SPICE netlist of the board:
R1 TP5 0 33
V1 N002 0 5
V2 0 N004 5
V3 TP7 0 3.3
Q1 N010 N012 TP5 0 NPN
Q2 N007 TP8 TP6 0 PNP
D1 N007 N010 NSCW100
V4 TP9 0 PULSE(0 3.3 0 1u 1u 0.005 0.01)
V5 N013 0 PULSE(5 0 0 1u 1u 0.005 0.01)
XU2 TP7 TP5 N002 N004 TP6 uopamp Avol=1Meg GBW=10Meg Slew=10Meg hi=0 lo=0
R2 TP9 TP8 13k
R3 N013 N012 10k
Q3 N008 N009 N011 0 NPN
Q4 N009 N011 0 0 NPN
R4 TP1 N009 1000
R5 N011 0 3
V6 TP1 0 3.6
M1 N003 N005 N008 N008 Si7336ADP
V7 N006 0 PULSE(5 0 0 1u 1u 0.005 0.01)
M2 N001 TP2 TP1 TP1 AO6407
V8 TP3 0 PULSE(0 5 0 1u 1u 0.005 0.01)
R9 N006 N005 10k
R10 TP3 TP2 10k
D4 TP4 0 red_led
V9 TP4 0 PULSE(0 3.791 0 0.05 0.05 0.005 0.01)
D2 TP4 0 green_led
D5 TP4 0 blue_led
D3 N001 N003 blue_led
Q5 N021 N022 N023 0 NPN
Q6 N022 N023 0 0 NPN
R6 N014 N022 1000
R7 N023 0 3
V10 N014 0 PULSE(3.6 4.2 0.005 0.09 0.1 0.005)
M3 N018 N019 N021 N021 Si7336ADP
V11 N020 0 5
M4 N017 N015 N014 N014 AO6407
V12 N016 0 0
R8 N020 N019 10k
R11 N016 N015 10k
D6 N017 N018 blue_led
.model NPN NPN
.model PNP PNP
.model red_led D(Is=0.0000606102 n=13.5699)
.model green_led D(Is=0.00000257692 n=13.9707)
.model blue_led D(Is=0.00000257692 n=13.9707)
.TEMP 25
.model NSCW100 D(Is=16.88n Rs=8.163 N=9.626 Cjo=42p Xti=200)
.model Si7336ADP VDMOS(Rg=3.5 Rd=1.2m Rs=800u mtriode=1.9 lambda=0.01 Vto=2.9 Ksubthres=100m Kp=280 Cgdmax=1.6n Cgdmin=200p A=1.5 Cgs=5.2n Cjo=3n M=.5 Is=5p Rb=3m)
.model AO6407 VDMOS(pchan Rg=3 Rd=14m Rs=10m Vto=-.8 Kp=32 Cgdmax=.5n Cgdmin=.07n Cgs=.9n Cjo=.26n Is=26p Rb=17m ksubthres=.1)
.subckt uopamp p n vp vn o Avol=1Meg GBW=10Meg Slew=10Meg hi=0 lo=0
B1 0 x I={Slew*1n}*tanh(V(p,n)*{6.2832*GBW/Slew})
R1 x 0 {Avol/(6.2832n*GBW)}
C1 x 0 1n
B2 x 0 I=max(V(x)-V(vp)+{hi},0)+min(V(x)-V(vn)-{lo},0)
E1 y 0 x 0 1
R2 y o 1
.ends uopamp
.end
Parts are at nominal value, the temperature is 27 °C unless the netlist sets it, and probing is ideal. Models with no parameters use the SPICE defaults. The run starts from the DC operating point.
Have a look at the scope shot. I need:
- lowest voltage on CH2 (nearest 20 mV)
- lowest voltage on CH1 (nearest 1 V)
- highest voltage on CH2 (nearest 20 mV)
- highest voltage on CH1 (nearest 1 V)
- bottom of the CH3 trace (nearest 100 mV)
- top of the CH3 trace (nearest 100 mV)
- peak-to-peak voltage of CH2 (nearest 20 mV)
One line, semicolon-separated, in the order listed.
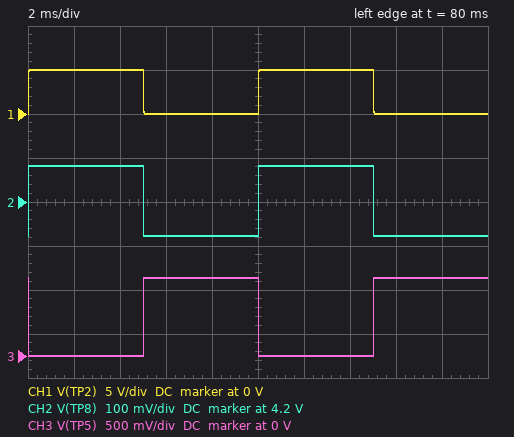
4.12 V; 0 V; 4.28 V; 5 V; 0 V; 900 mV; 160 mV
